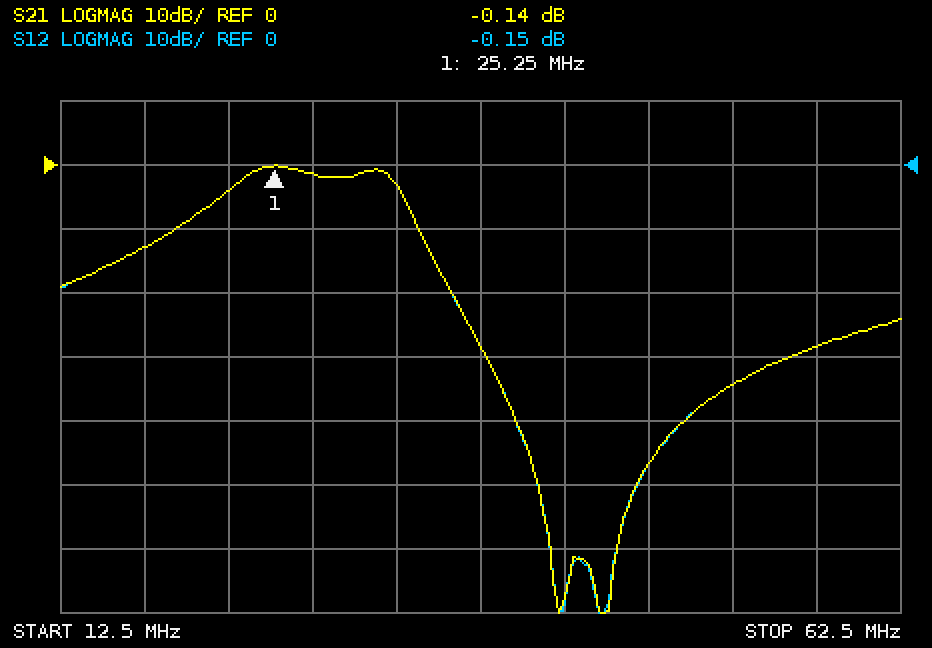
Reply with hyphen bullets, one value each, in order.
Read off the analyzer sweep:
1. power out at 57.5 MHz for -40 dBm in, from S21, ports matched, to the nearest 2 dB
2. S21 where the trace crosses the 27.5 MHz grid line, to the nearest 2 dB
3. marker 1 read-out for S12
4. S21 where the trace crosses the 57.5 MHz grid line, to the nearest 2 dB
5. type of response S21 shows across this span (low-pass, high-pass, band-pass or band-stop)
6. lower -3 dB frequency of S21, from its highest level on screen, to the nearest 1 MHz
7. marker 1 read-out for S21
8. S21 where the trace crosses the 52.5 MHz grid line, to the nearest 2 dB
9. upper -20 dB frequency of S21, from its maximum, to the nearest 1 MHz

- -68 dBm
- -2 dB
- -0.15 dB
- -28 dB
- band-pass
- 23 MHz
- -0.14 dB
- -34 dB
- 36 MHz
